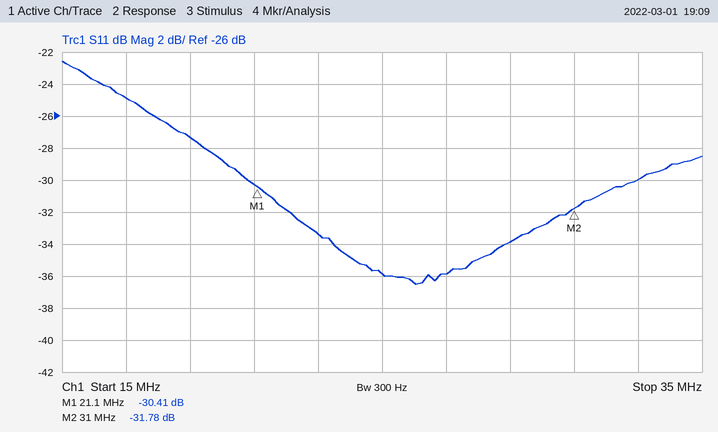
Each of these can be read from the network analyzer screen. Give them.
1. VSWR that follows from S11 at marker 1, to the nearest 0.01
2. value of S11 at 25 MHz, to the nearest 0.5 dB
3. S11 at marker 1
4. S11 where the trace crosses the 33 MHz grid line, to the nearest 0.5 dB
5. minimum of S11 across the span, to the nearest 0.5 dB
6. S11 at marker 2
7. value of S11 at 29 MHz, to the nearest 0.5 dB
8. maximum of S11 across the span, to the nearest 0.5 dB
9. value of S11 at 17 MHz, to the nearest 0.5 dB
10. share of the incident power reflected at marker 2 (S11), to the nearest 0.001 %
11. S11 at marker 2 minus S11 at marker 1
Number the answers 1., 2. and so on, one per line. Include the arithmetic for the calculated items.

1. (1 + 0.0302)/(1 − 0.0302) ≈ 1.06
2. -36.0 dB
3. -30.41 dB
4. -30.0 dB
5. -36.5 dB
6. -31.78 dB
7. -34.0 dB
8. -22.5 dB
9. -25.0 dB
10. 10^(-31.78/10) ≈ 0.066 %
11. -31.78 − (-30.41) = -1.37 dB
